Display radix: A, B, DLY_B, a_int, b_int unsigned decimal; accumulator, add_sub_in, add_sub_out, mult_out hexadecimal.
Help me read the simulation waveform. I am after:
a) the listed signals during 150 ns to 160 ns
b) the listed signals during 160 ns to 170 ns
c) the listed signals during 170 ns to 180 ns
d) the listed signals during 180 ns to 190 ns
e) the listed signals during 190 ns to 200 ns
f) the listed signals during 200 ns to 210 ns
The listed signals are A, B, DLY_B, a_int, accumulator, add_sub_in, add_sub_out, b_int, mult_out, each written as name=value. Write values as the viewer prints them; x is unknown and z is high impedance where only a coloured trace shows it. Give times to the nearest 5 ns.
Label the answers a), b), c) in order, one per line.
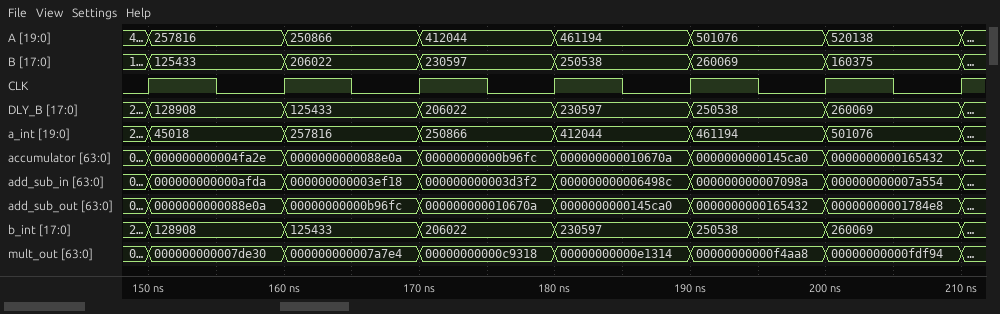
a) A=257816, B=125433, DLY_B=128908, a_int=45018, accumulator=000000000004fa2e, add_sub_in=000000000000afda, add_sub_out=0000000000088e0a, b_int=128908, mult_out=000000000007de30
b) A=250866, B=206022, DLY_B=125433, a_int=257816, accumulator=0000000000088e0a, add_sub_in=000000000003ef18, add_sub_out=00000000000b96fc, b_int=125433, mult_out=000000000007a7e4
c) A=412044, B=230597, DLY_B=206022, a_int=250866, accumulator=00000000000b96fc, add_sub_in=000000000003d3f2, add_sub_out=000000000010670a, b_int=206022, mult_out=00000000000c9318
d) A=461194, B=250538, DLY_B=230597, a_int=412044, accumulator=000000000010670a, add_sub_in=000000000006498c, add_sub_out=0000000000145ca0, b_int=230597, mult_out=00000000000e1314
e) A=501076, B=260069, DLY_B=250538, a_int=461194, accumulator=0000000000145ca0, add_sub_in=000000000007098a, add_sub_out=0000000000165432, b_int=250538, mult_out=00000000000f4aa8
f) A=520138, B=160375, DLY_B=260069, a_int=501076, accumulator=0000000000165432, add_sub_in=000000000007a554, add_sub_out=00000000001784e8, b_int=260069, mult_out=00000000000fdf94
